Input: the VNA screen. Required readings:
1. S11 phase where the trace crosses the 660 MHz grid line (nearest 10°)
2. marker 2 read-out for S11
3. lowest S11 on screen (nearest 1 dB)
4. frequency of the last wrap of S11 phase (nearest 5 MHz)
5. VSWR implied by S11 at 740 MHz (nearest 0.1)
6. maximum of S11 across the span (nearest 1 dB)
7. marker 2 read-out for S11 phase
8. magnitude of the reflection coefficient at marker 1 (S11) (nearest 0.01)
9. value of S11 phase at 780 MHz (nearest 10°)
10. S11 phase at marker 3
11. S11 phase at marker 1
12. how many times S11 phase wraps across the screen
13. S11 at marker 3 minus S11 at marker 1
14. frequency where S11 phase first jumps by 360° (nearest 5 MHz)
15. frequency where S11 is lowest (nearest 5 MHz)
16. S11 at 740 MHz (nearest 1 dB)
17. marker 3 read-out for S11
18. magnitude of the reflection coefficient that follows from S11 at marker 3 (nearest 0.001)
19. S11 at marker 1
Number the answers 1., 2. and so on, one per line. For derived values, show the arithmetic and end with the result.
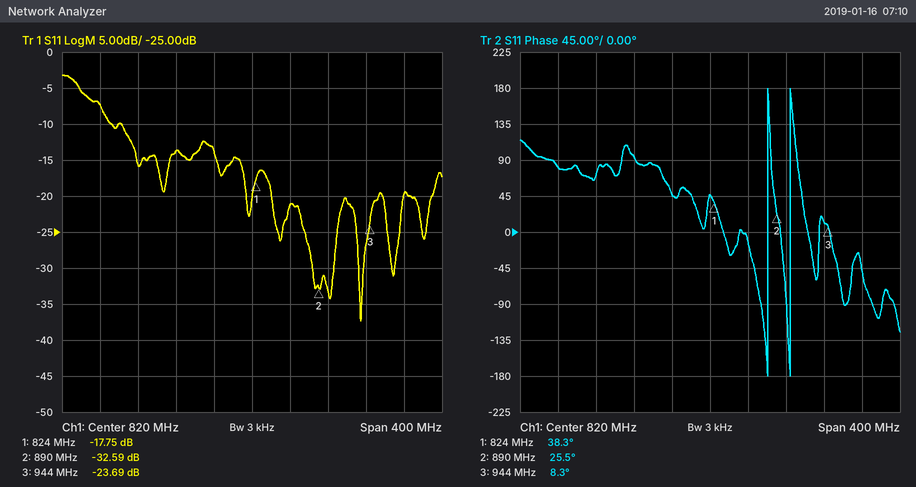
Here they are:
1. 80°
2. -32.59 dB
3. -37 dB
4. 905 MHz
5. |Γ| = 10^(-14/20) = 0.1995; VSWR = (1 + 0.1995)/(1 − 0.1995) ≈ 1.5
6. -3 dB
7. 25.5°
8. 10^(-17.75/20) ≈ 0.13
9. 50°
10. 8.3°
11. 38.3°
12. 2
13. -23.69 − (-17.75) = -5.94 dB
14. 880 MHz
15. 935 MHz
16. -14 dB
17. -23.69 dB
18. 10^(-23.69/20) ≈ 0.065
19. -17.75 dB
